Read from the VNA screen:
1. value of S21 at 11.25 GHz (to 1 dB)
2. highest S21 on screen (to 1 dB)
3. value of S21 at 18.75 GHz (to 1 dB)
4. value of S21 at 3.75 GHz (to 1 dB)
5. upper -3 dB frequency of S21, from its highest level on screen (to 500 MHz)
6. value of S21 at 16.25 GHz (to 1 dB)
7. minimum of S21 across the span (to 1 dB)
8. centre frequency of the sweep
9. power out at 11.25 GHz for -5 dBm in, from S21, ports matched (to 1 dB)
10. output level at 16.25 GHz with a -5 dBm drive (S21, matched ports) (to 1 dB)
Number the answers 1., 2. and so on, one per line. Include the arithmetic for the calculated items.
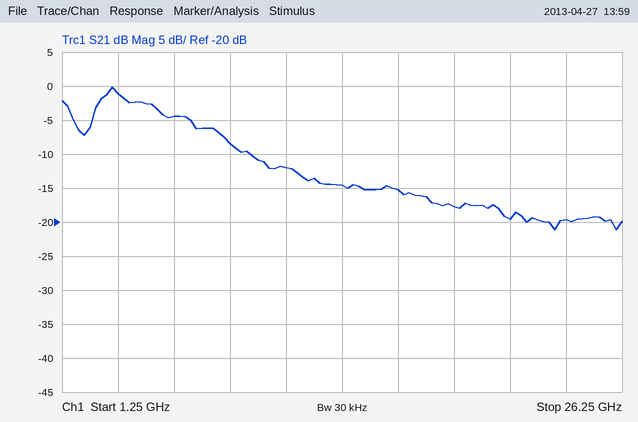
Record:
1. -12 dB
2. 0 dB
3. -18 dB
4. -1 dB
5. 5.5 GHz
6. -15 dB
7. -21 dB
8. 13.75 GHz
9. -5 dBm + (-12 dB) = -17 dBm
10. -5 dBm + (-15 dB) = -20 dBm
